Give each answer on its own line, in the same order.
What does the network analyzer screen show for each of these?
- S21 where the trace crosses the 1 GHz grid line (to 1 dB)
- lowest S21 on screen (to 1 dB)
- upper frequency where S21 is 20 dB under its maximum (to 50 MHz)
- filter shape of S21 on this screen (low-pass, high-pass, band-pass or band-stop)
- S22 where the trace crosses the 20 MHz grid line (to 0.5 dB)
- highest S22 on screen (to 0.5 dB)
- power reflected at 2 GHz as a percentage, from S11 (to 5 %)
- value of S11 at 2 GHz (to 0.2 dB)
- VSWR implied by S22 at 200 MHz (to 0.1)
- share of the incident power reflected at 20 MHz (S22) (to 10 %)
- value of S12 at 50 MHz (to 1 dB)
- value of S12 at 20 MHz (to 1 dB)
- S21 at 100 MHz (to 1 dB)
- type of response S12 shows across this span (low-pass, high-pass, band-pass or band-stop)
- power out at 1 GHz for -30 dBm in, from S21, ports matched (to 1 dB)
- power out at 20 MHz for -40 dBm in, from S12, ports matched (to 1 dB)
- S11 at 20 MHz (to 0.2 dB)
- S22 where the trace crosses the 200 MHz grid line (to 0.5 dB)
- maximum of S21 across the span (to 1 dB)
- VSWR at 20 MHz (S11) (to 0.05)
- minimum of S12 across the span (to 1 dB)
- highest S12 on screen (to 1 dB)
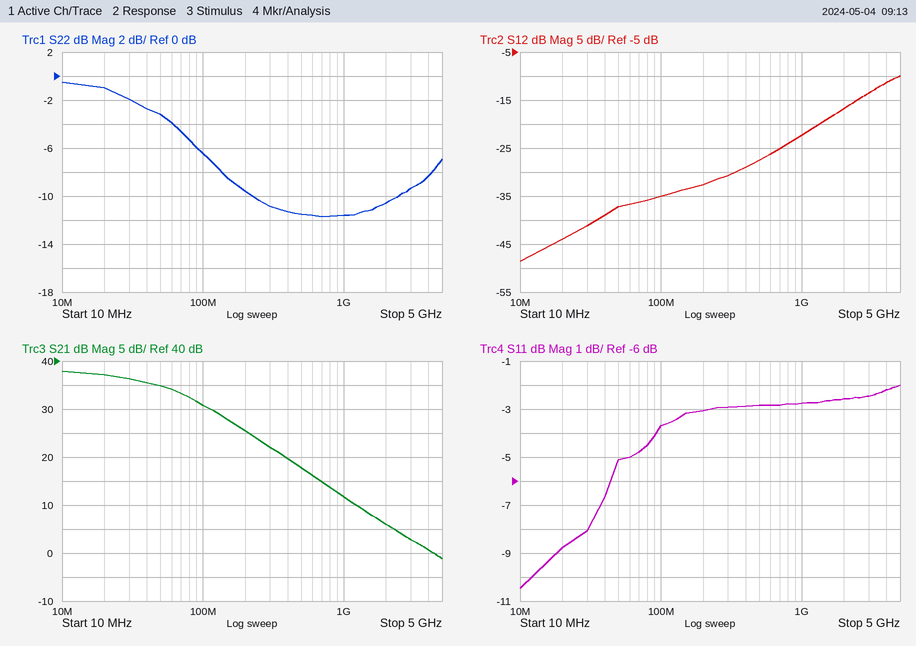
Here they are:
12 dB
-1 dB
500 MHz
low-pass
-1.0 dB
-0.5 dB
55 %
-2.6 dB
2.0
80 %
-37 dB
-44 dB
31 dB
high-pass
-18 dBm
-84 dBm
-8.8 dB
-9.5 dB
38 dB
2.15
-49 dB
-10 dB
